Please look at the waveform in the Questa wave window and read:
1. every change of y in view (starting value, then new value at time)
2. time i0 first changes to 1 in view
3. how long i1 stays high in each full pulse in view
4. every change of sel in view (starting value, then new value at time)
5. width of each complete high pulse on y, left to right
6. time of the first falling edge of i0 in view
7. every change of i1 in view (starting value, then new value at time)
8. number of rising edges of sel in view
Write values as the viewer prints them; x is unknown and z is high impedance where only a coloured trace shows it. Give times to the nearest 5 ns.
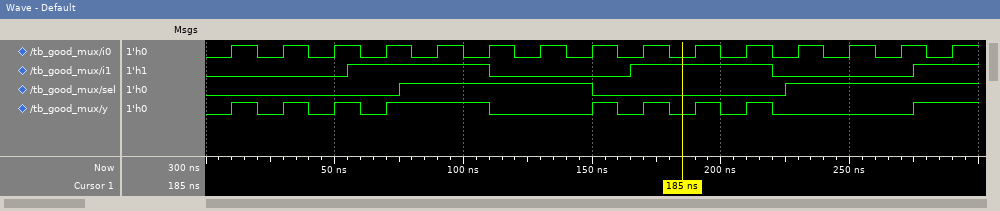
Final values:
0, 1 at 10 ns, 0 at 20 ns, 1 at 30 ns, 0 at 40 ns, 1 at 50 ns, 0 at 60 ns, 1 at 70 ns, 0 at 110 ns, 1 at 150 ns, 0 at 160 ns, 1 at 170 ns, 0 at 180 ns, 1 at 190 ns, 0 at 200 ns, 1 at 210 ns, 0 at 220 ns, 1 at 275 ns
10 ns
55 ns, 55 ns
0, 1 at 75 ns, 0 at 150 ns, 1 at 225 ns
10 ns, 10 ns, 10 ns, 40 ns, 10 ns, 10 ns, 10 ns, 10 ns
20 ns
0, 1 at 55 ns, 0 at 110 ns, 1 at 165 ns, 0 at 220 ns, 1 at 275 ns
2
